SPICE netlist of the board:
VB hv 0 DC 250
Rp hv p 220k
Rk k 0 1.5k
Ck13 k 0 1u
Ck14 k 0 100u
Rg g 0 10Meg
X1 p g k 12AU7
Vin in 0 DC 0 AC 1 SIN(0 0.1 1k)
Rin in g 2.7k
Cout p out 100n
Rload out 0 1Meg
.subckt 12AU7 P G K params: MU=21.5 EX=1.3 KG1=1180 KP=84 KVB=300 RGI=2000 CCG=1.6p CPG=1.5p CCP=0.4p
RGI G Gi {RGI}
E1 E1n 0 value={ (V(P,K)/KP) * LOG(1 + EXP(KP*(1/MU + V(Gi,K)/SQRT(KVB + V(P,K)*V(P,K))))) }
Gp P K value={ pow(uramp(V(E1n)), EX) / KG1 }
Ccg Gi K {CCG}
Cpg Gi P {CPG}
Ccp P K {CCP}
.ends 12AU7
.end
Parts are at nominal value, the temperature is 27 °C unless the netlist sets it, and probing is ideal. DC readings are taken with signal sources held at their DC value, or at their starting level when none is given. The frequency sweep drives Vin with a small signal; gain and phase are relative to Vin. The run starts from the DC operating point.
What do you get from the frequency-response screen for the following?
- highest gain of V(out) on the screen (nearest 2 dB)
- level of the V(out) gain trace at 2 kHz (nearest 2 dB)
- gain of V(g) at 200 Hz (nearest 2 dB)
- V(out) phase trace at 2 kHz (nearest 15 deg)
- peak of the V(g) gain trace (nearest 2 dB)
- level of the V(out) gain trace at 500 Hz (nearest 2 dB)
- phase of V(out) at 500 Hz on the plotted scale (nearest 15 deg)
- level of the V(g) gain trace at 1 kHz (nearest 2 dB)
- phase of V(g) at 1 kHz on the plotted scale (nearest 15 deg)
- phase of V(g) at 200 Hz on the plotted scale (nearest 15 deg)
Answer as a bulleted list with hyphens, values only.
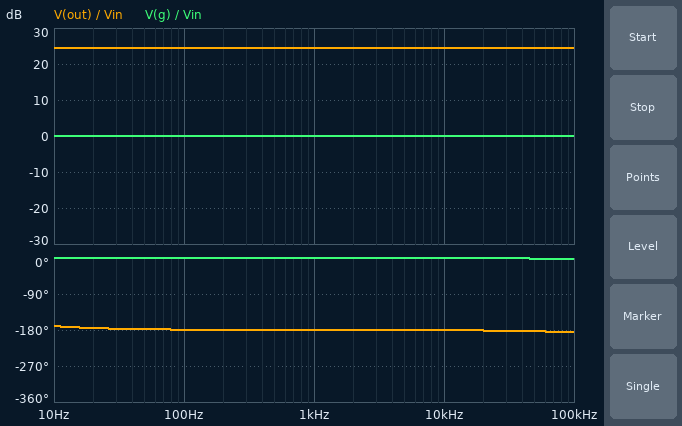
- 24 dB
- 24 dB
- 0 dB
- -180 deg
- 0 dB
- 24 dB
- -180 deg
- 0 dB
- 0 deg
- 0 deg
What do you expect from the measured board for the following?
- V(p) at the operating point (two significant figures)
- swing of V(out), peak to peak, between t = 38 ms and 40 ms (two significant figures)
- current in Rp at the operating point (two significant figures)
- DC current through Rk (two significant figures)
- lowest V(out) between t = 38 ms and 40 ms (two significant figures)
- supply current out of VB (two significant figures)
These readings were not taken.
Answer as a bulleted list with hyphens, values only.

- 50 V
- 3.4 V
- 910 µA
- 910 µA
- -1.7 V
- 910 µA
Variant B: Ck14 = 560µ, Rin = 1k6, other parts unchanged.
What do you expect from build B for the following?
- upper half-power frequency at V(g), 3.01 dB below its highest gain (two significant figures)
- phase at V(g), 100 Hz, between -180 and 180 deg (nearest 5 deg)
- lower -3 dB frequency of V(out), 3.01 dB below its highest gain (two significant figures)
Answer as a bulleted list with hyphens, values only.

- 3.6 MHz
- 0 deg
- 1.6 Hz
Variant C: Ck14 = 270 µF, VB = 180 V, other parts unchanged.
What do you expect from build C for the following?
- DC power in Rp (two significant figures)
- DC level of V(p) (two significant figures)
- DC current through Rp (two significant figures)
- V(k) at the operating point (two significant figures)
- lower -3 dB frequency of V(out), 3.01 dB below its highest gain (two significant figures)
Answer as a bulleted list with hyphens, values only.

- 94 mW
- 36 V
- 650 µA
- 980 mV
- 1.6 Hz
